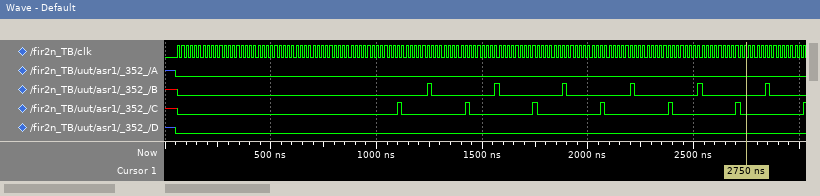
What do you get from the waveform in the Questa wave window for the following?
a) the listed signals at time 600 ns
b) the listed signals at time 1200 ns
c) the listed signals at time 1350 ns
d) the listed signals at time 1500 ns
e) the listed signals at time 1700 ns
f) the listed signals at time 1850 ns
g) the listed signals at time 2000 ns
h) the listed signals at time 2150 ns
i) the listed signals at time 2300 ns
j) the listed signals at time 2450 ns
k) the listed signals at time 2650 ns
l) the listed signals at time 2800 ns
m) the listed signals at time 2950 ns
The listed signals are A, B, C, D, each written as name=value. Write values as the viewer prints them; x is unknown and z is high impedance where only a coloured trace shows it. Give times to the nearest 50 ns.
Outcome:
A=0, B=0, C=0, D=0
A=0, B=0, C=0, D=0
A=0, B=0, C=0, D=0
A=0, B=0, C=0, D=0
A=0, B=0, C=0, D=0
A=0, B=0, C=0, D=0
A=0, B=0, C=0, D=0
A=0, B=0, C=0, D=0
A=0, B=0, C=0, D=0
A=0, B=0, C=0, D=0
A=0, B=0, C=0, D=0
A=0, B=0, C=0, D=0
A=0, B=0, C=0, D=0
